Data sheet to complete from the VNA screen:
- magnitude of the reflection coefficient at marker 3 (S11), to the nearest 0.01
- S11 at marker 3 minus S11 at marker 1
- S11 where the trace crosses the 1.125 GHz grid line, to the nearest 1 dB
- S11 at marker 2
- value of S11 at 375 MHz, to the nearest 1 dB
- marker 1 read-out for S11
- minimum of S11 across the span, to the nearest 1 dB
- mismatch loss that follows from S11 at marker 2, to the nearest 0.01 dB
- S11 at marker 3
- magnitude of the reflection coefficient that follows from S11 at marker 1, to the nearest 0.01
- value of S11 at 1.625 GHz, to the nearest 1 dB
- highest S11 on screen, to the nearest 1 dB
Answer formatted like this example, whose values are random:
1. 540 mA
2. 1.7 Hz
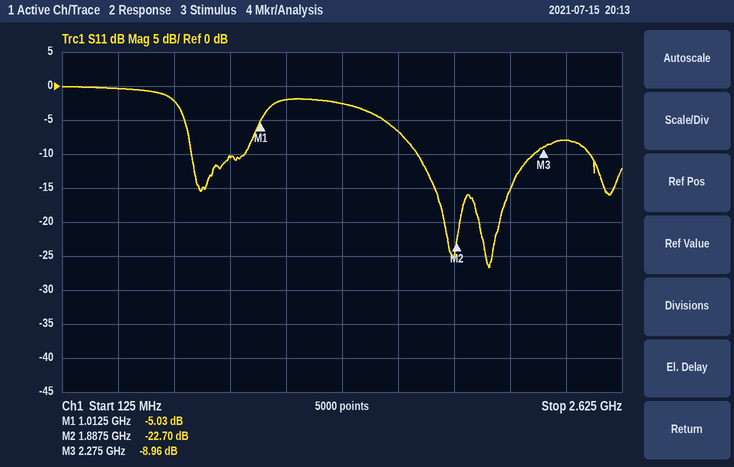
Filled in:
1. 0.36
2. -3.93 dB
3. -2 dB
4. -22.70 dB
5. 0 dB
6. -5.03 dB
7. -27 dB
8. 0.02 dB
9. -8.96 dB
10. 0.56
11. -7 dB
12. 0 dB
